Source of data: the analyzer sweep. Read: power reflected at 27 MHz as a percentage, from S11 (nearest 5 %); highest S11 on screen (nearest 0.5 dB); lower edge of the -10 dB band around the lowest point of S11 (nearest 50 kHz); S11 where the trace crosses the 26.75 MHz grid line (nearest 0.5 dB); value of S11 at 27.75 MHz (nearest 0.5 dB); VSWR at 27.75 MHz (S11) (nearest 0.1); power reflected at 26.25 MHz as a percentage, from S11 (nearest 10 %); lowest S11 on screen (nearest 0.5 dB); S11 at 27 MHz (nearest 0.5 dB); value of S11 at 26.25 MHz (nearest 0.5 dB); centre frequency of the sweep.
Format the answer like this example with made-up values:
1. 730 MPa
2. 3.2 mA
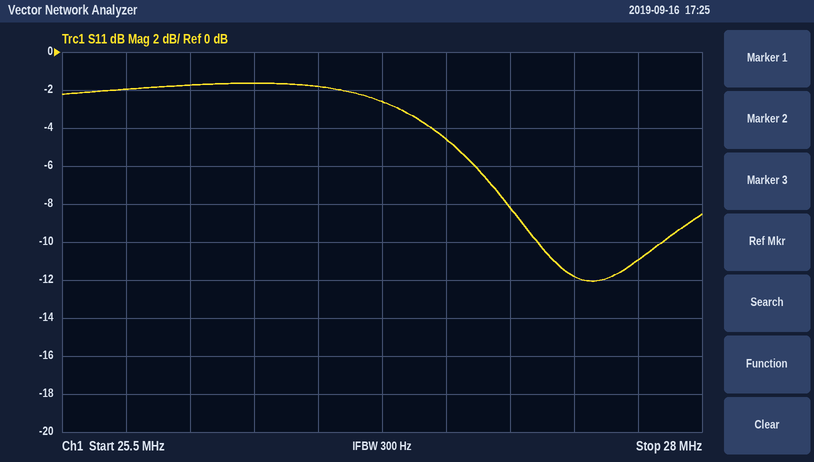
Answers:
1. 35 %
2. -1.5 dB
3. 27.35 MHz
4. -2.5 dB
5. -11.0 dB
6. 1.8
7. 70 %
8. -12.0 dB
9. -4.5 dB
10. -1.5 dB
11. 26.75 MHz
